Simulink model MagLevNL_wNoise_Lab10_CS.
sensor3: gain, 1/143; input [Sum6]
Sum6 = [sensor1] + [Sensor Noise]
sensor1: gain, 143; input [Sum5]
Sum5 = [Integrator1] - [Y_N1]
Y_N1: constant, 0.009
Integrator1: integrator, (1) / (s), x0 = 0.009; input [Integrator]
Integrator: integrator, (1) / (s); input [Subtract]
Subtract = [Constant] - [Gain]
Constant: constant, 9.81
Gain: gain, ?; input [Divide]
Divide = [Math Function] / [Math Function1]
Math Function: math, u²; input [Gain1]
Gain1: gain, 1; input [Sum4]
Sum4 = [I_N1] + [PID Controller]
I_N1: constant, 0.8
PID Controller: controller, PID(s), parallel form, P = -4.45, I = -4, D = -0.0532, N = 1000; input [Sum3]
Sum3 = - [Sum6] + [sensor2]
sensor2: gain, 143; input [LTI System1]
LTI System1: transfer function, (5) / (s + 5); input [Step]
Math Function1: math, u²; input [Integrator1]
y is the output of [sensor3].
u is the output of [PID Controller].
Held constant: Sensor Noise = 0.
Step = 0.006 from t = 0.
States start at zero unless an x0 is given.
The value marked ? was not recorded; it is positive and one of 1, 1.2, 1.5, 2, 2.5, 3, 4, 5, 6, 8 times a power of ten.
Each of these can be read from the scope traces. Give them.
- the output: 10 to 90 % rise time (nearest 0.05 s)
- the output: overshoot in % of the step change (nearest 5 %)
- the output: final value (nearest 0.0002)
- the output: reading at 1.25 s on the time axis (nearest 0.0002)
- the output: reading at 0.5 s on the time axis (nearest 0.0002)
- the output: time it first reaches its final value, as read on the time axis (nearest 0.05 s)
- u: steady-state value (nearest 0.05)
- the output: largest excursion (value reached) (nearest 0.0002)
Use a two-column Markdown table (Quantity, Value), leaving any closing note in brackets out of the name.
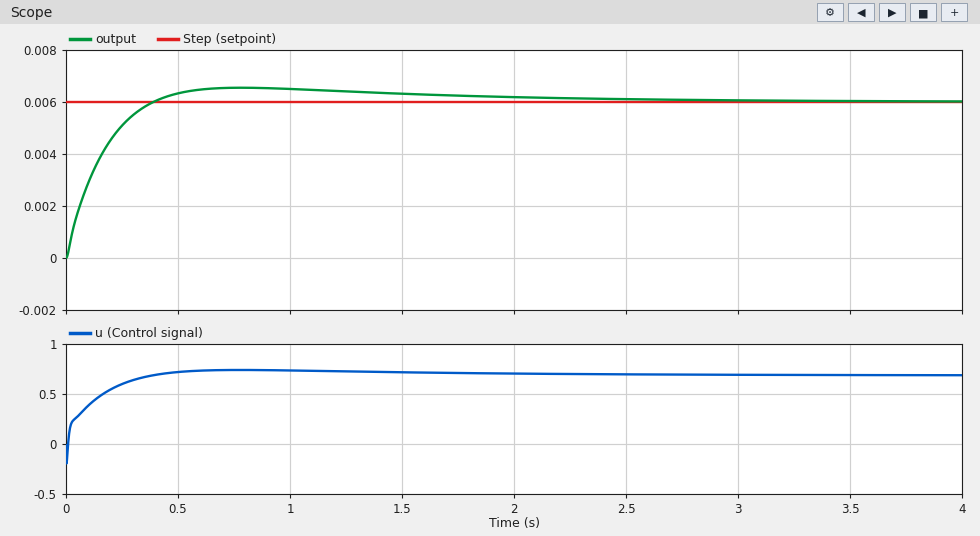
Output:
| Quantity | Value |
|---|---|
| the output: 10 to 90 % rise time | 0.25 s |
| the output: overshoot in % of the step change | 10 % |
| the output: final value | 0.0060 |
| the output: reading at 1.25 s on the time axis | 0.0064 |
| the output: reading at 0.5 s on the time axis | 0.0064 |
| the output: time it first reaches its final value, as read on the time axis | 0.40 s |
| u: steady-state value | 0.70 |
| the output: largest excursion (value reached) | 0.0066 |
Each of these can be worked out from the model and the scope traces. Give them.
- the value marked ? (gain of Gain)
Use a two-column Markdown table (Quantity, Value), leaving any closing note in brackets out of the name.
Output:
| Quantity | Value |
|---|---|
| the value marked ? | 0.001 |
